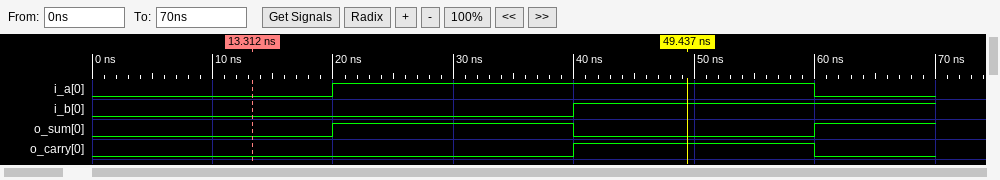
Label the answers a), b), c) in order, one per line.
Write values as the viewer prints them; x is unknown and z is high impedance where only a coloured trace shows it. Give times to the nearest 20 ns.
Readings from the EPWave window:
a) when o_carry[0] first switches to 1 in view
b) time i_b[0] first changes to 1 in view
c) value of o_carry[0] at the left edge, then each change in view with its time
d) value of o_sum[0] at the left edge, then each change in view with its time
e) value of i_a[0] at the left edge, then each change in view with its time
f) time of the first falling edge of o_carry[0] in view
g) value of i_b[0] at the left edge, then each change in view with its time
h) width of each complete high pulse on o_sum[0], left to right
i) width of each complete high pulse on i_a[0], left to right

a) 40 ns
b) 40 ns
c) 0, 1 at 40 ns, 0 at 60 ns
d) 0, 1 at 20 ns, 0 at 40 ns, 1 at 60 ns
e) 0, 1 at 20 ns, 0 at 60 ns
f) 60 ns
g) 0, 1 at 40 ns
h) 20 ns
i) 40 ns
